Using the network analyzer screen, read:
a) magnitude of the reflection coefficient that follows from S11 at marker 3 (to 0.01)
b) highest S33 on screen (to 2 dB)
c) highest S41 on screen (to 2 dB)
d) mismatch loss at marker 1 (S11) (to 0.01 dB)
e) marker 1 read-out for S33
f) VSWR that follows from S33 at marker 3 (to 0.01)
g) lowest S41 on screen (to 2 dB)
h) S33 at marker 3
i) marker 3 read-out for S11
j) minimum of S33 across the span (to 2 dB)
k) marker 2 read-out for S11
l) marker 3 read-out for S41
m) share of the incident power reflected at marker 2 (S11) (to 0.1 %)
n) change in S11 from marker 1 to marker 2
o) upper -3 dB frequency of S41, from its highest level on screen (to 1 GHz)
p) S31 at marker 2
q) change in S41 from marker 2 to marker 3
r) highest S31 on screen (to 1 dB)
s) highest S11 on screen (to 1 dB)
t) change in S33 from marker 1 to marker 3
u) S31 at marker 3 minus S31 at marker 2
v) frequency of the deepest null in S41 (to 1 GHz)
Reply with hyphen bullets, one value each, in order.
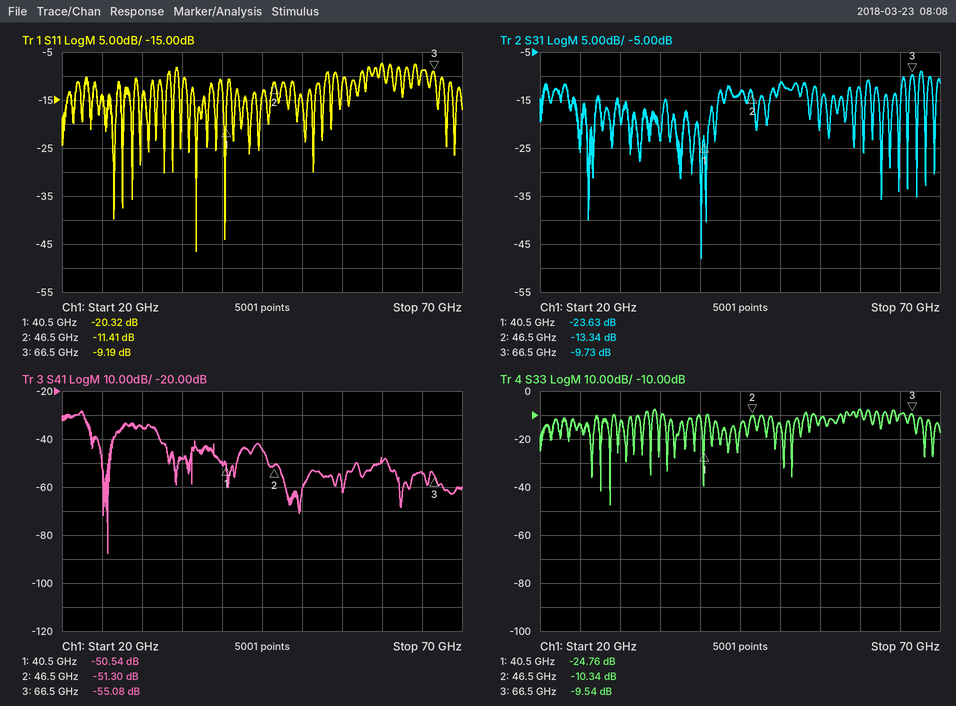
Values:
- 0.35
- -8 dB
- -28 dB
- 0.04 dB
- -24.76 dB
- 2.00
- -88 dB
- -9.54 dB
- -9.19 dB
- -48 dB
- -11.41 dB
- -55.08 dB
- 7.2 %
- 8.91 dB
- 23 GHz
- -13.34 dB
- -3.78 dB
- -9 dB
- -7 dB
- 15.22 dB
- 3.61 dB
- 26 GHz
